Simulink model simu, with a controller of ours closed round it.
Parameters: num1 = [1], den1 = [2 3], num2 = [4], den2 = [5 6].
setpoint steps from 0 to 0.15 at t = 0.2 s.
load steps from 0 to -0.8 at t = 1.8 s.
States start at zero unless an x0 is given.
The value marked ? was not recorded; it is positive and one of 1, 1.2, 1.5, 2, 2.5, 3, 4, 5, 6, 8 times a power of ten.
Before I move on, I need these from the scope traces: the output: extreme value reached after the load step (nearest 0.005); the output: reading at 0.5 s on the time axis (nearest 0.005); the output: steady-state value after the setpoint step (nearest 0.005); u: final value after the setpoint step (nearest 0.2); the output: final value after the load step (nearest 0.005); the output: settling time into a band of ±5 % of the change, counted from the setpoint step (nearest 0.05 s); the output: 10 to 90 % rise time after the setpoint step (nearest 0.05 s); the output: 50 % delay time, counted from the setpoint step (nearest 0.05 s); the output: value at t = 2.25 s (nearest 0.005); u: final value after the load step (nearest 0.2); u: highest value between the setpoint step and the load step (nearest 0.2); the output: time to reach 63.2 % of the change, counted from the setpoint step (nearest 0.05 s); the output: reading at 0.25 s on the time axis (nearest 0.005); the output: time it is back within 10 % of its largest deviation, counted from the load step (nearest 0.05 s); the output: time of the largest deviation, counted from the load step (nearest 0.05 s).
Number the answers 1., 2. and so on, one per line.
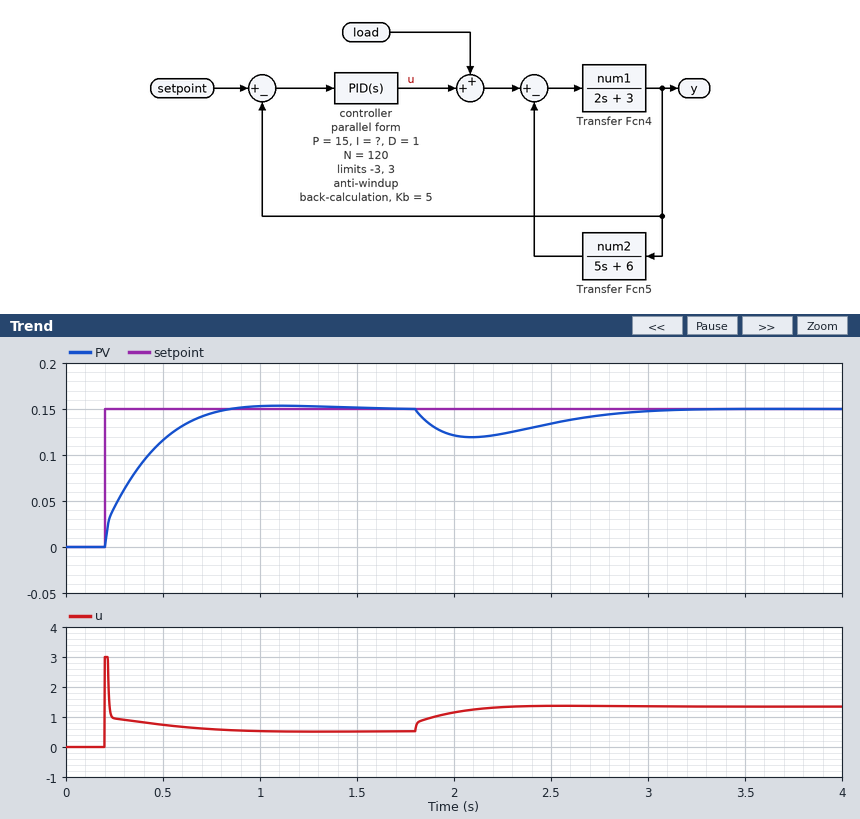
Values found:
1. 0.120
2. 0.115
3. 0.150
4. 0.6
5. 0.150
6. 0.50 s
7. 0.40 s
8. 0.15 s
9. 0.125
10. 1.4
11. 3.0
12. 0.20 s
13. 0.045
14. 1.15 s
15. 0.30 s
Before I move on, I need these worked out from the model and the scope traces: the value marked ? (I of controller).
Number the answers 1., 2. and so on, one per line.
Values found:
1. 40
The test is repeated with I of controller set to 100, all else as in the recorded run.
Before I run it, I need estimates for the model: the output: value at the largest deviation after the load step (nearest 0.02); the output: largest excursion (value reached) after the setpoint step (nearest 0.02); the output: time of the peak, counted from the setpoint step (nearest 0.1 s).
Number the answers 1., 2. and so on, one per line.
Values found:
1. 0.12
2. 0.18
3. 0.5 s
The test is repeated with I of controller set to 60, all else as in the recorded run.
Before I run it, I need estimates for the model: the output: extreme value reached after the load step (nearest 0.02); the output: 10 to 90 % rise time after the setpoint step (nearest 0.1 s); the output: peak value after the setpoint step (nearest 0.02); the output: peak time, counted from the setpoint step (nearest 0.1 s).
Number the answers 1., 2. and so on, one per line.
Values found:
1. 0.12
2. 0.3 s
3. 0.16
4. 0.7 s
